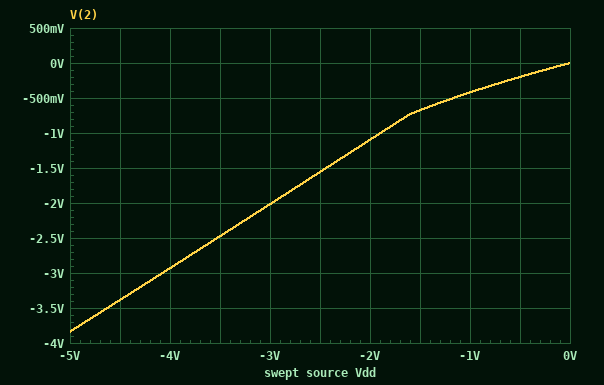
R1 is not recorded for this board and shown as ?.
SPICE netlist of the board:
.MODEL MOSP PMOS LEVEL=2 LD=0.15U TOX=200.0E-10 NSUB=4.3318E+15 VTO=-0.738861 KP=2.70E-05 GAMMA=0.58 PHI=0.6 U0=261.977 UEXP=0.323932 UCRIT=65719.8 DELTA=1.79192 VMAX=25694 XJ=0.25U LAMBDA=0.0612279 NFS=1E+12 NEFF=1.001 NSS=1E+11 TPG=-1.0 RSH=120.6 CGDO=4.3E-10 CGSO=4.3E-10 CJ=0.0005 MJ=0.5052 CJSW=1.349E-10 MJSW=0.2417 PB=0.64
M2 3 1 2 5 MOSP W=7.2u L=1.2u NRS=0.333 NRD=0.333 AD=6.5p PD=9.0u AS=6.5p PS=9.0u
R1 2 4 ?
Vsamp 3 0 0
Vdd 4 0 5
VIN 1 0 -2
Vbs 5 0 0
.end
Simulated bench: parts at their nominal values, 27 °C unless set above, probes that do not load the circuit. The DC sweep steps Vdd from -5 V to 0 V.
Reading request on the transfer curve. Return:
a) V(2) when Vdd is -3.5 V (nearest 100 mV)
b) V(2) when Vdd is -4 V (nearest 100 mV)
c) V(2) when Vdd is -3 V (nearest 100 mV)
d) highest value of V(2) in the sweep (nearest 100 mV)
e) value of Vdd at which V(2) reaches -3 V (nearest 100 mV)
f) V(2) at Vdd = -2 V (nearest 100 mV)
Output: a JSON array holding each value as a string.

["-2.5 V", "-2.9 V", "-2.0 V", "0 V", "-4.1 V", "-1.1 V"]
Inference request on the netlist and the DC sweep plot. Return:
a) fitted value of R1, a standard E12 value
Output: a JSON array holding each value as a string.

["8.2 kΩ"]
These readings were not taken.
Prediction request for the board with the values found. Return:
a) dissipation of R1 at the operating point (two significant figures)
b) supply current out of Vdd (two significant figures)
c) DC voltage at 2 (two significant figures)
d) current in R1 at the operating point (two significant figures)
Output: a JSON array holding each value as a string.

["2.3 mW", "530 µA", "650 mV", "530 µA"]
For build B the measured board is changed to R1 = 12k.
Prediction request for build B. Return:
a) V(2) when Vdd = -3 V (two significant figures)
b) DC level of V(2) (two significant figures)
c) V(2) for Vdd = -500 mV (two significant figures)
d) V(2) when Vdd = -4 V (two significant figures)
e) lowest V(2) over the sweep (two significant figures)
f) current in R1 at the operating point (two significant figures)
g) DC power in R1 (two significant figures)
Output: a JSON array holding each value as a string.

["-1.6 V", "630 mV", "-150 mV", "-2.5 V", "-3.4 V", "360 µA", "1.6 mW"]
